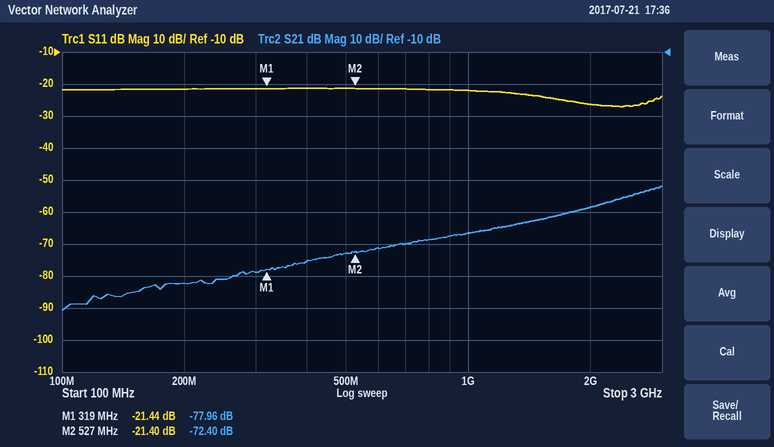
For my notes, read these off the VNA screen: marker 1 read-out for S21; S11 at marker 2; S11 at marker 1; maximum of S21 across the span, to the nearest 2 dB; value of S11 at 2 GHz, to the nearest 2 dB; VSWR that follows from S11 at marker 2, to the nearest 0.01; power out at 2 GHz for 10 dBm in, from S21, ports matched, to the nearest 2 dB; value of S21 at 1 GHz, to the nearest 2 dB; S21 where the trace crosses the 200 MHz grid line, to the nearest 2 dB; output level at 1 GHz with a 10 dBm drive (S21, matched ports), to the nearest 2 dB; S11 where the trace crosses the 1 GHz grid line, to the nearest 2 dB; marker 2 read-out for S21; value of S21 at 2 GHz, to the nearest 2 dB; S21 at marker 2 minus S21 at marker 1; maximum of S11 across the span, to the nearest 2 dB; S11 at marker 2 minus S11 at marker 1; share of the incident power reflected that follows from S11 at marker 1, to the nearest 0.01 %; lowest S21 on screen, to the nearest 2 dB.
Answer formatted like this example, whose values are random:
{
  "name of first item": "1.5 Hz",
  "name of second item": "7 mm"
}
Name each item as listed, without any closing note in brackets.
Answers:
{
  "marker 1 read-out for S21": "-77.96 dB",
  "S11 at marker 2": "-21.40 dB",
  "S11 at marker 1": "-21.44 dB",
  "maximum of S21 across the span, to the nearest 2 dB": "-52 dB",
  "value of S11 at 2 GHz, to the nearest 2 dB": "-26 dB",
  "VSWR that follows from S11 at marker 2, to the nearest 0.01": "1.19",
  "power out at 2 GHz for 10 dBm in, from S21, ports matched, to the nearest 2 dB": "-48 dBm",
  "value of S21 at 1 GHz, to the nearest 2 dB": "-66 dB",
  "S21 where the trace crosses the 200 MHz grid line, to the nearest 2 dB": "-82 dB",
  "output level at 1 GHz with a 10 dBm drive (S21, matched ports), to the nearest 2 dB": "-56 dBm",
  "S11 where the trace crosses the 1 GHz grid line, to the nearest 2 dB": "-22 dB",
  "marker 2 read-out for S21": "-72.40 dB",
  "value of S21 at 2 GHz, to the nearest 2 dB": "-58 dB",
  "S21 at marker 2 minus S21 at marker 1": "5.56 dB",
  "maximum of S11 across the span, to the nearest 2 dB": "-22 dB",
  "S11 at marker 2 minus S11 at marker 1": "0.04 dB",
  "share of the incident power reflected that follows from S11 at marker 1, to the nearest 0.01 %": "0.72 %",
  "lowest S21 on screen, to the nearest 2 dB": "-90 dB"
}
